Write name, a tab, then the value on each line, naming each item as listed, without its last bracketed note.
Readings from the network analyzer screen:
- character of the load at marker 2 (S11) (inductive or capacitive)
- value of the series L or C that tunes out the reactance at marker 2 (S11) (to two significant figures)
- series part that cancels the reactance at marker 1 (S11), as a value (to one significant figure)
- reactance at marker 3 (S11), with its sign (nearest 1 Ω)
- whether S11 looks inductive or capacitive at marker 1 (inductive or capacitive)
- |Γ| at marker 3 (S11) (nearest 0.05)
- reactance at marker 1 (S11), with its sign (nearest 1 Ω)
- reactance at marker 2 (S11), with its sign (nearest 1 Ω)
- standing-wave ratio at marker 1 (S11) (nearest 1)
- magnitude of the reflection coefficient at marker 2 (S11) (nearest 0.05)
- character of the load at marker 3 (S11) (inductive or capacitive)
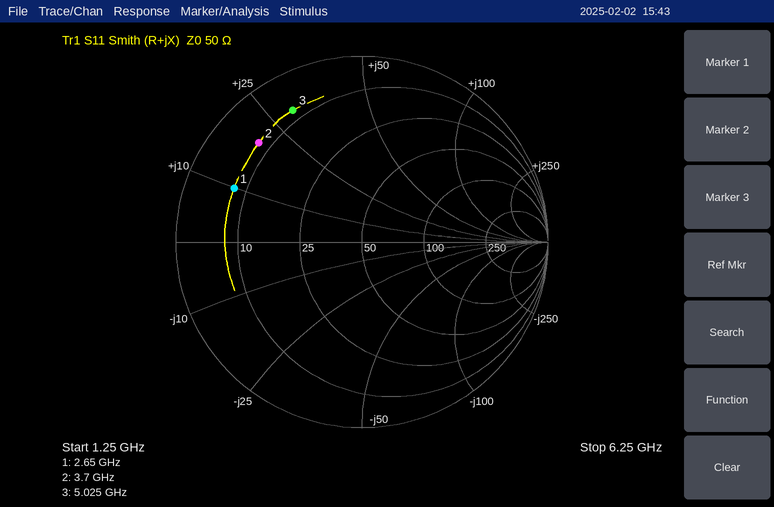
character of the load at marker 2 (S11)	inductive
value of the series L or C that tunes out the reactance at marker 2 (S11)	2.2 pF
series part that cancels the reactance at marker 1 (S11), as a value	6 pF
reactance at marker 3 (S11), with its sign	+30 Ω
whether S11 looks inductive or capacitive at marker 1	inductive
|Γ| at marker 3 (S11)	0.80
reactance at marker 1 (S11), with its sign	+10 Ω
reactance at marker 2 (S11), with its sign	+20 Ω
standing-wave ratio at marker 1 (S11)	7
magnitude of the reflection coefficient at marker 2 (S11)	0.75
character of the load at marker 3 (S11)	inductive
